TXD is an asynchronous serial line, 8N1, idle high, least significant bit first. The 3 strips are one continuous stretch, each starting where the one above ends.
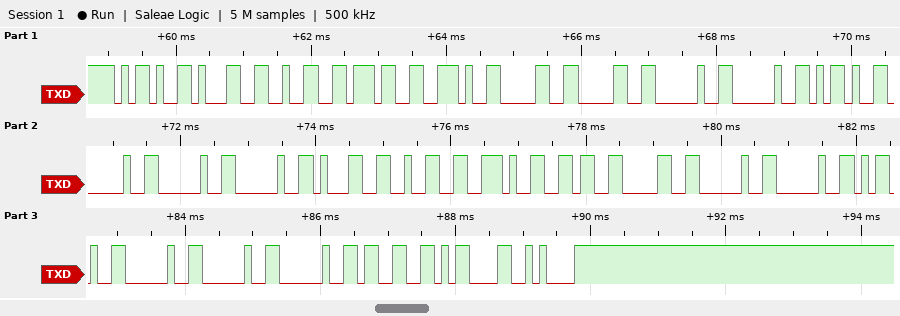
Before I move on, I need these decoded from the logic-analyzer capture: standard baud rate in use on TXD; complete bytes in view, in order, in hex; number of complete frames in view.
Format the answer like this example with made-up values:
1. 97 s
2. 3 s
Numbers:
1. 9600 baud
2. 2D 31 32 37 2E 30 30 20 20 2D 20 20 20 31 32 2E 36 30 20 20 2D 20 20 20 33 0D 0A
3. 27
